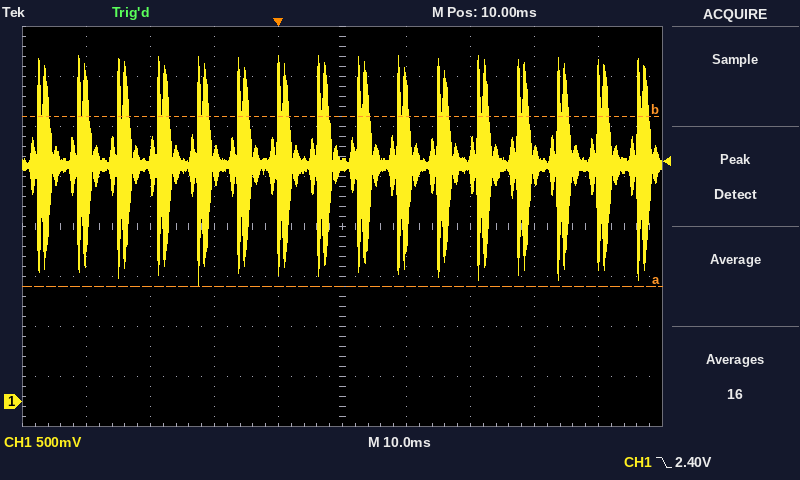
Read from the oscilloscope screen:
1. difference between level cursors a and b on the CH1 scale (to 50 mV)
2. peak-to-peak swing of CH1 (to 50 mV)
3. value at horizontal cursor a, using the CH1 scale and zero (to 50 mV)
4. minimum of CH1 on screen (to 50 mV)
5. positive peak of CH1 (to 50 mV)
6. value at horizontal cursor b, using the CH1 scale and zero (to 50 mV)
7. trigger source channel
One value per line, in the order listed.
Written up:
1.70 V
2.30 V
1.15 V
1.15 V
3.45 V
2.85 V
CH1
